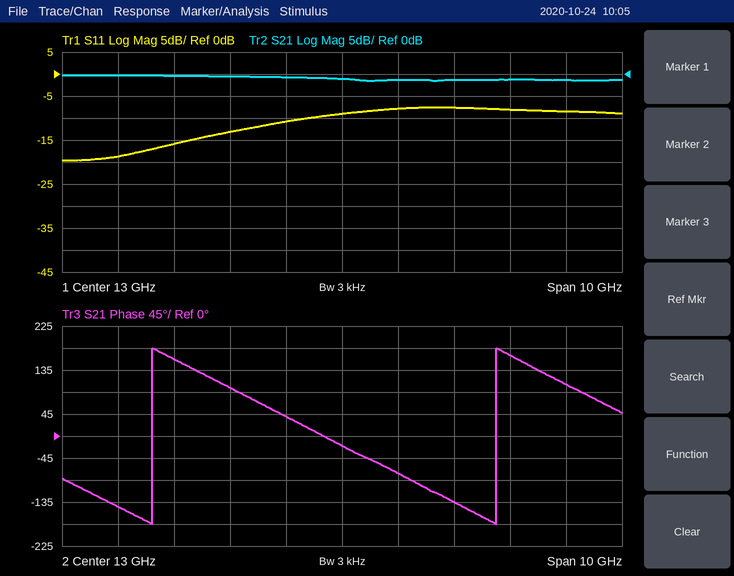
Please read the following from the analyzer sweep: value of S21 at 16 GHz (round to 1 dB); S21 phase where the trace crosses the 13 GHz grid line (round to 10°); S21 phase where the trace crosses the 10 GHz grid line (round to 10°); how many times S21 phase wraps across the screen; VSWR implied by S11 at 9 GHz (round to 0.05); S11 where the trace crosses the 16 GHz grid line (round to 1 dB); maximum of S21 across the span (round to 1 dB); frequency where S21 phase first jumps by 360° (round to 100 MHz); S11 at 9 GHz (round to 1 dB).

-1 dB
-20°
160°
2
1.25
-8 dB
0 dB
9.6 GHz
-19 dB
